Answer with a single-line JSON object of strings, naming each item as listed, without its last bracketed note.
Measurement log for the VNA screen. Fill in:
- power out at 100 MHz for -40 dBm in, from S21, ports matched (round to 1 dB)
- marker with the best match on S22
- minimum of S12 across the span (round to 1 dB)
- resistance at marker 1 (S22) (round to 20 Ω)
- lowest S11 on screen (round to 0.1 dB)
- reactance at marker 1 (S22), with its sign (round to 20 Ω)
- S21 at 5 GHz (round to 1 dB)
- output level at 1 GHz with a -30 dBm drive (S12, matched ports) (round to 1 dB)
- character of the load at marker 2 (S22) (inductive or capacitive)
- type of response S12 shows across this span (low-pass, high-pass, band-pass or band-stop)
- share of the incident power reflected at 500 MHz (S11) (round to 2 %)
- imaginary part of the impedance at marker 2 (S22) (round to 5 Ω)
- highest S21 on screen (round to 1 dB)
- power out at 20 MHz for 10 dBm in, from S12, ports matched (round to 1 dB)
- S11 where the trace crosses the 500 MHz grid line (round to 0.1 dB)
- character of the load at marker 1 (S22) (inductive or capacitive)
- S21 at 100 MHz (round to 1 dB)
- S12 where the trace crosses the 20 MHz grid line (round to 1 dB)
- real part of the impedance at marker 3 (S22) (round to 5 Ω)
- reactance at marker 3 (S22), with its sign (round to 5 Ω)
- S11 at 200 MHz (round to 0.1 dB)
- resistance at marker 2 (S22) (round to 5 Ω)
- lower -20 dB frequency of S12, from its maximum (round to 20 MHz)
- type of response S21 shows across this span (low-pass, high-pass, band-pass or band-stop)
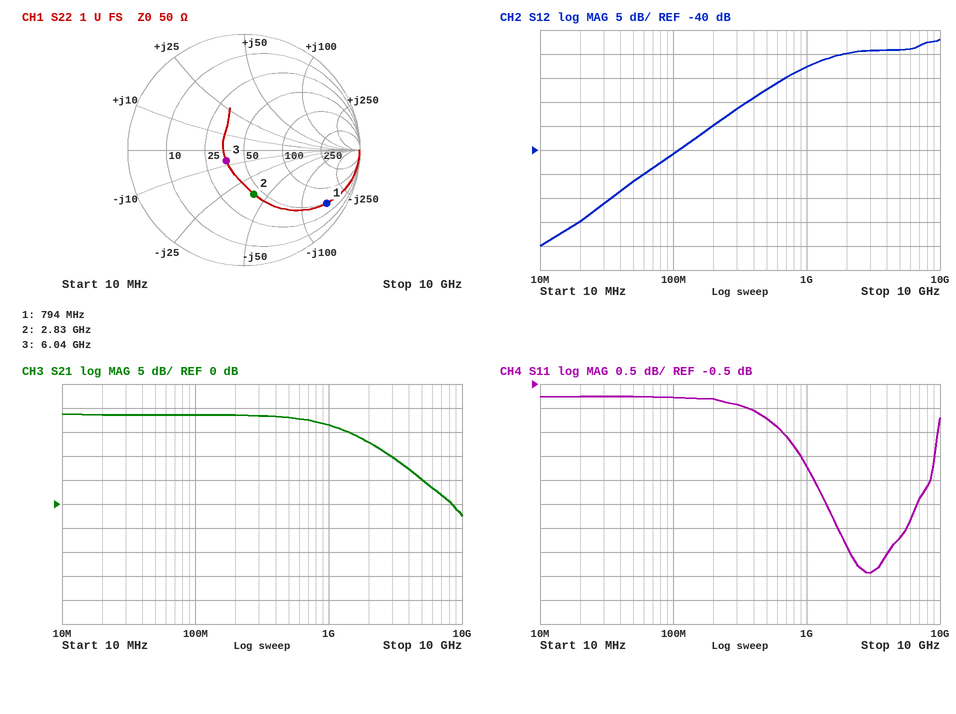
{"power out at 100 MHz for -40 dBm in, from S21, ports matched": "-21 dBm", "marker with the best match on S22": "marker 3", "minimum of S12 across the span": "-60 dB", "resistance at marker 1 (S22)": "40 Ω", "lowest S11 on screen": "-4.4 dB", "reactance at marker 1 (S22), with its sign": "-160 Ω", "S21 at 5 GHz": "5 dB", "output level at 1 GHz with a -30 dBm drive (S12, matched ports)": "-53 dBm", "character of the load at marker 2 (S22)": "capacitive", "type of response S12 shows across this span": "high-pass", "share of the incident power reflected at 500 MHz (S11)": "76 %", "imaginary part of the impedance at marker 2 (S22)": "-40 Ω", "highest S21 on screen": "19 dB", "power out at 20 MHz for 10 dBm in, from S12, ports matched": "-45 dBm", "S11 where the trace crosses the 500 MHz grid line": "-1.2 dB", "character of the load at marker 1 (S22)": "capacitive", "S21 at 100 MHz": "19 dB", "S12 where the trace crosses the 20 MHz grid line": "-55 dB", "real part of the impedance at marker 3 (S22)": "35 Ω", "reactance at marker 3 (S22), with its sign": "-5 Ω", "S11 at 200 MHz": "-0.8 dB", "resistance at marker 2 (S22)": "45 Ω", "lower -20 dB frequency of S12, from its maximum": "160 MHz", "type of response S21 shows across this span": "low-pass"}
